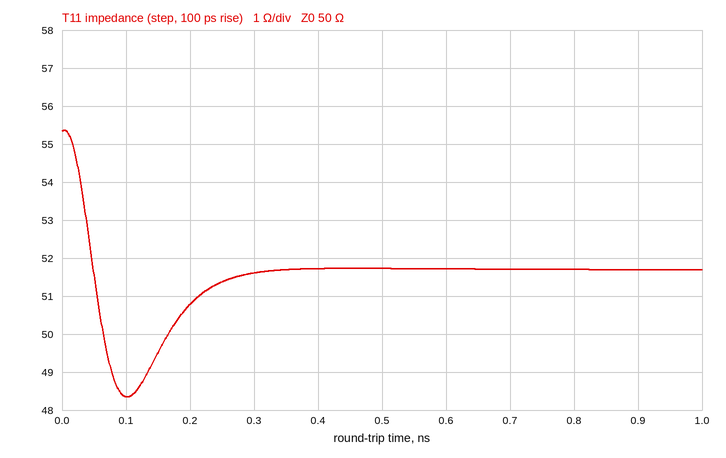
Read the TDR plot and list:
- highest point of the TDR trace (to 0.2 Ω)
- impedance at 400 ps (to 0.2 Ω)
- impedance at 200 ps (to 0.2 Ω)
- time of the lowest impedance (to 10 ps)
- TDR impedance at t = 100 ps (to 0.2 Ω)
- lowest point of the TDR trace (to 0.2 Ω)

55.4 Ω
51.8 Ω
50.8 Ω
100 ps
48.4 Ω
48.4 Ω
